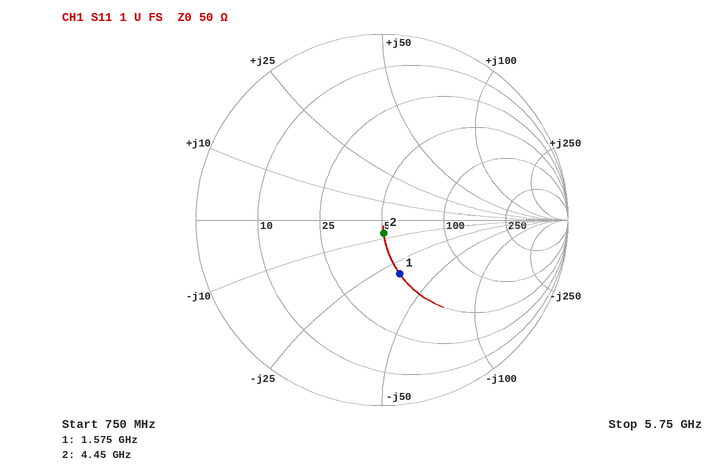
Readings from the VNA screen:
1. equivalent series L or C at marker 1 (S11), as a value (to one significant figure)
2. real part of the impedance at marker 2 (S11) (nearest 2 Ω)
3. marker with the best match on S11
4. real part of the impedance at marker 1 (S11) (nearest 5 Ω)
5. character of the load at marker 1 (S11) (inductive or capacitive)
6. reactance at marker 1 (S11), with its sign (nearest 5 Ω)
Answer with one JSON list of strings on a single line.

["3 pF", "50 Ω", "marker 2", "50 Ω", "capacitive", "-30 Ω"]
